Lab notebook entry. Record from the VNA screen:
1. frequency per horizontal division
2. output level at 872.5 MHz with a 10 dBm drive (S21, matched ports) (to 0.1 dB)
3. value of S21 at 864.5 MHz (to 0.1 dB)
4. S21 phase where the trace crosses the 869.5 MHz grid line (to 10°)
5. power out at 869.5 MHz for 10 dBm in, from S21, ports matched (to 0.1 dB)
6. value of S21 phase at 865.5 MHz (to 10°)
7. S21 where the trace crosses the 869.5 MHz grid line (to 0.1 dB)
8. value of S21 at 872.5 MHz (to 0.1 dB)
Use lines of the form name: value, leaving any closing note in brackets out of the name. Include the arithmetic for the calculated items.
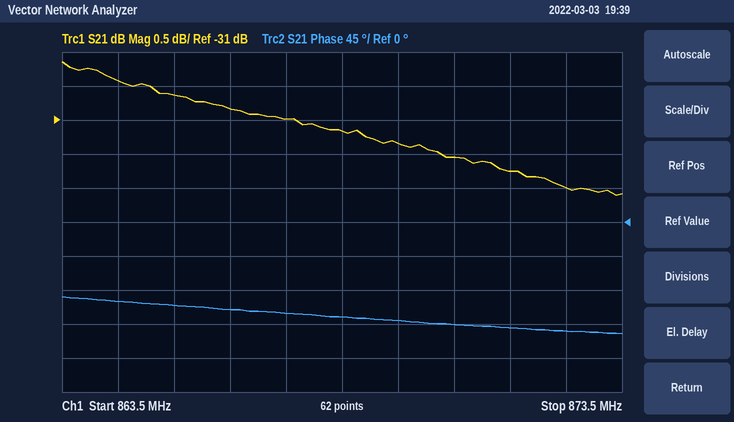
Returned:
frequency per horizontal division: 1 MHz
output level at 872.5 MHz with a 10 dBm drive (S21, matched ports): 10 dBm + (-32.0 dB) = -22.0 dBm
value of S21 at 864.5 MHz: -30.4 dB
S21 phase where the trace crosses the 869.5 MHz grid line: -130°
power out at 869.5 MHz for 10 dBm in, from S21, ports matched: 10 dBm + (-31.3 dB) = -21.3 dBm
value of S21 phase at 865.5 MHz: -110°
S21 where the trace crosses the 869.5 MHz grid line: -31.3 dB
value of S21 at 872.5 MHz: -32.0 dB
